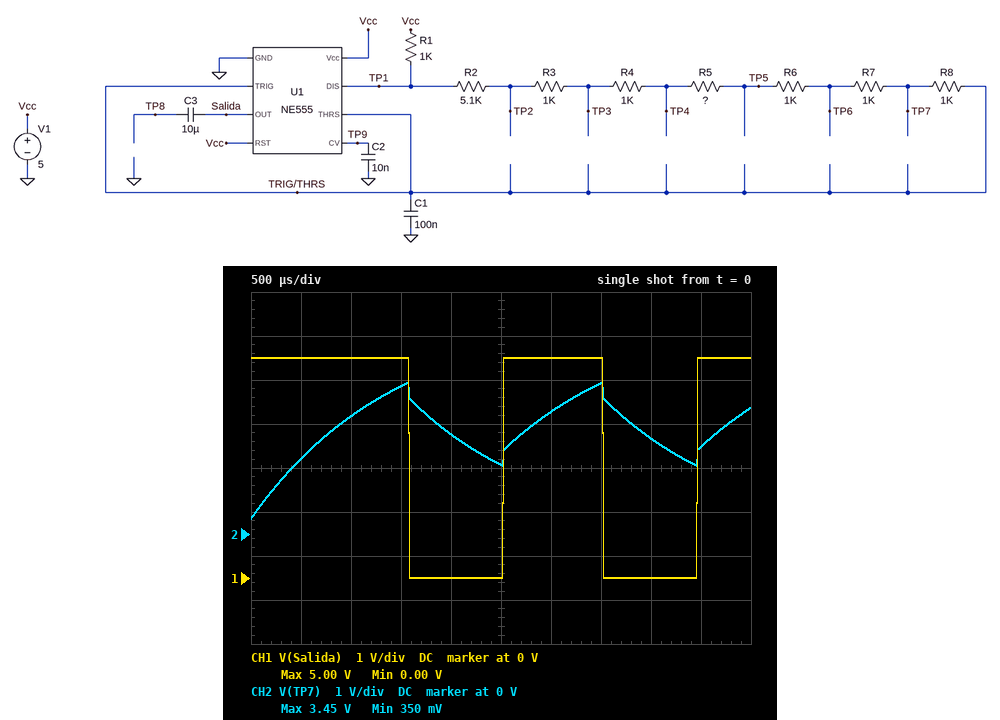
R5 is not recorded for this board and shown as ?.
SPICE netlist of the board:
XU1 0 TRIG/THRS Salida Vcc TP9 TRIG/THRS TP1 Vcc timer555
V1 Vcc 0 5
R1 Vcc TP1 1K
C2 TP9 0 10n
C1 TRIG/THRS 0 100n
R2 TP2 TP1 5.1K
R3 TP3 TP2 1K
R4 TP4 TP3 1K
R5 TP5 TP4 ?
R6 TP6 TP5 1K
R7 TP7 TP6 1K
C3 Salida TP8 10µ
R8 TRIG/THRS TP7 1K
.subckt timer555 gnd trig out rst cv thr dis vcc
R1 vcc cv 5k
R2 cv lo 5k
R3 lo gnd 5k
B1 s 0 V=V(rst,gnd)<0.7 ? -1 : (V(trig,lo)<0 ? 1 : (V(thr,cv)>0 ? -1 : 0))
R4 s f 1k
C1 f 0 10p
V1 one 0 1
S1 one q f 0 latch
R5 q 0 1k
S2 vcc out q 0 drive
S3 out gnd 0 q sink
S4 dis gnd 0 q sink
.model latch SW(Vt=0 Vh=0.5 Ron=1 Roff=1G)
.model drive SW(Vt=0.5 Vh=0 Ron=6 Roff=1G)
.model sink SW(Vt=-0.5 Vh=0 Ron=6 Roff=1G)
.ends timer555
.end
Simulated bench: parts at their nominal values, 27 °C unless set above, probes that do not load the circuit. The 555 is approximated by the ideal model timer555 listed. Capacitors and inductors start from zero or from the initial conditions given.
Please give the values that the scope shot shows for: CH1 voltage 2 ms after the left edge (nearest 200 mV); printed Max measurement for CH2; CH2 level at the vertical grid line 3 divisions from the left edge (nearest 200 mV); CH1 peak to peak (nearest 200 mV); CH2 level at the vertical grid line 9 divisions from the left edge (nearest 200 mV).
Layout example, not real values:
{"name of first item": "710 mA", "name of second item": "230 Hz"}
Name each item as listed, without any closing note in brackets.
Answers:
{"CH1 voltage 2 ms after the left edge": "0 V", "printed Max measurement for CH2": "3.45 V", "CH2 level at the vertical grid line 3 divisions from the left edge": "3.4 V", "CH1 peak to peak": "5.0 V", "CH2 level at the vertical grid line 9 divisions from the left edge": "2.0 V"}
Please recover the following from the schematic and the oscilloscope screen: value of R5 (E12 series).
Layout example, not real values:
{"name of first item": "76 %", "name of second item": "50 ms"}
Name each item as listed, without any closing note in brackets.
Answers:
{"value of R5": "3.3 kΩ"}
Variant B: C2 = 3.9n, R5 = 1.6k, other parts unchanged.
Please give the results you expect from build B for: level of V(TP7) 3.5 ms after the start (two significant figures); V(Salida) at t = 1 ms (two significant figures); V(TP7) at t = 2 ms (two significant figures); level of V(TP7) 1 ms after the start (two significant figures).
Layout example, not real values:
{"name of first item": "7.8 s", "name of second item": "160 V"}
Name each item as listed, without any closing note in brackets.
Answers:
{"level of V(TP7) 3.5 ms after the start": "2.2 V", "V(Salida) at t = 1 ms": "5.0 V", "V(TP7) at t = 2 ms": "1.8 V", "level of V(TP7) 1 ms after the start": "2.9 V"}
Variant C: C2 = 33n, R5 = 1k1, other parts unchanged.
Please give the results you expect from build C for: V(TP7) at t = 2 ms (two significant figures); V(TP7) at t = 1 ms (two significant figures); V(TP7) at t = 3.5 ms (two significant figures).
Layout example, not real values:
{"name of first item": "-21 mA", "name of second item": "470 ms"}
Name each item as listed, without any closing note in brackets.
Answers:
{"V(TP7) at t = 2 ms": "1.7 V", "V(TP7) at t = 1 ms": "3.0 V", "V(TP7) at t = 3.5 ms": "1.9 V"}
